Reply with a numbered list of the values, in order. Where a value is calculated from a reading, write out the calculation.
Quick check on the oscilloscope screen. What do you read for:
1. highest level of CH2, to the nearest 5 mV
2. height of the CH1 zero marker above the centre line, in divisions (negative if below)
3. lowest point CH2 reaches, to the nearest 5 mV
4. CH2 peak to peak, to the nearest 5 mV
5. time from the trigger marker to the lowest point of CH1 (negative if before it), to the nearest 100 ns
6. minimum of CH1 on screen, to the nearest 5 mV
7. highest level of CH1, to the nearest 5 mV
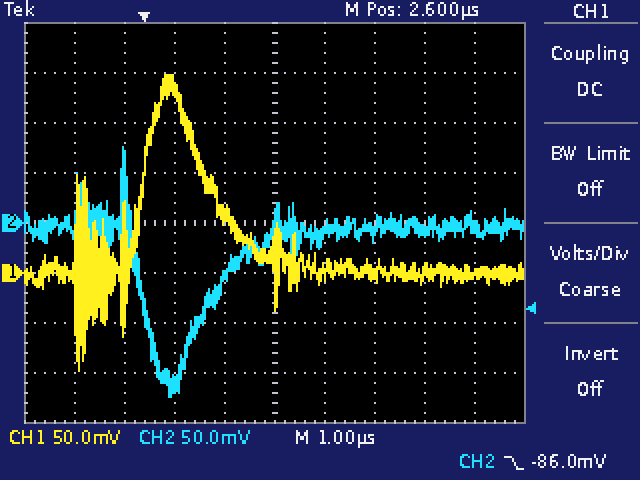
1. 75 mV
2. -1.0 div
3. -175 mV
4. 75 mV − (-175 mV) = 250 mV
5. -1.3 µs
6. -100 mV
7. 200 mV
